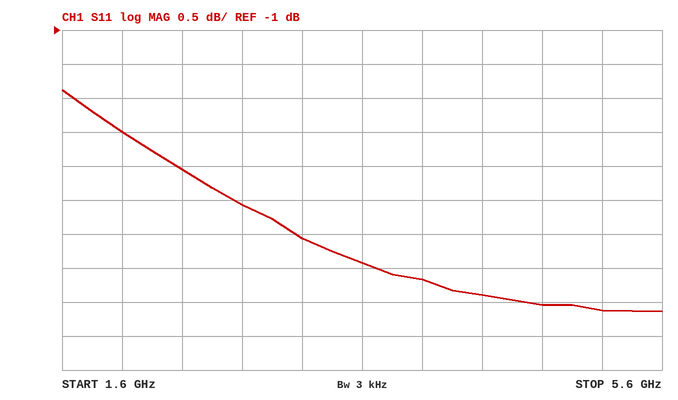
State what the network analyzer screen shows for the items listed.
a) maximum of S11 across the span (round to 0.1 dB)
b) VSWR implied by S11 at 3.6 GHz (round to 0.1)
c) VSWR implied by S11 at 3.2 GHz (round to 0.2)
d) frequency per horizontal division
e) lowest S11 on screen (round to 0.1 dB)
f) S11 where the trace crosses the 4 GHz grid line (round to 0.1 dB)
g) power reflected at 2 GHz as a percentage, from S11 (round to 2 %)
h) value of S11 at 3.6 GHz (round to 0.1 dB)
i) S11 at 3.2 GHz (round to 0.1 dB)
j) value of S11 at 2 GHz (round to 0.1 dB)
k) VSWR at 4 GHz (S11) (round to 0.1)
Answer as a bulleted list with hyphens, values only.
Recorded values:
- -1.9 dB
- 4.0
- 4.4
- 400 MHz
- -5.1 dB
- -4.7 dB
- 56 %
- -4.4 dB
- -4.1 dB
- -2.5 dB
- 3.8
